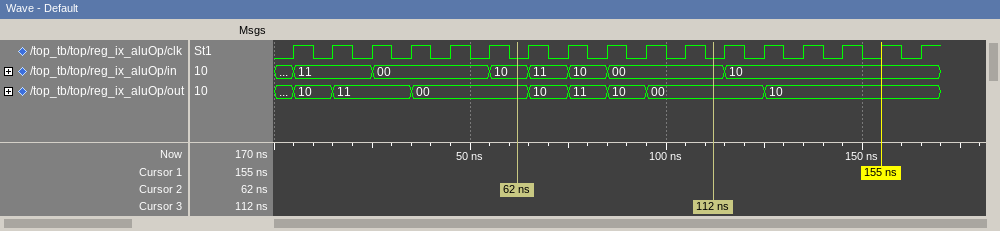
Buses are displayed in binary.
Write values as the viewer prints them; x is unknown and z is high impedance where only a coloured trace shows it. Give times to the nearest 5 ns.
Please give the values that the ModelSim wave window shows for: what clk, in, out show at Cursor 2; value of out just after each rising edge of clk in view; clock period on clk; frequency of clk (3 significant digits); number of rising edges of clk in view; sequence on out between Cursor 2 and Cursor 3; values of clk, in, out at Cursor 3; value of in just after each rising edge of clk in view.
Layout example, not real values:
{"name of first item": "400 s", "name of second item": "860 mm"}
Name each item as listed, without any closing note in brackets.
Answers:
{"what clk, in, out show at Cursor 2": "clk=0, in=10, out=00", "value of out just after each rising edge of clk in view": "10, 11, 11, 00, 00, 00, 10, 11, 10, 00, 00, 00, 10, 10, 10, 10, 10", "clock period on clk": "10 ns", "frequency of clk": "100 MHz", "number of rising edges of clk in view": "17", "sequence on out between Cursor 2 and Cursor 3": "00, 10, 11, 10, 00", "values of clk, in, out at Cursor 3": "clk=0, in=00, out=00", "value of in just after each rising edge of clk in view": "11, 11, 00, 00, 00, 10, 11, 10, 00, 00, 00, 10, 10, 10, 10, 10, 10"}
